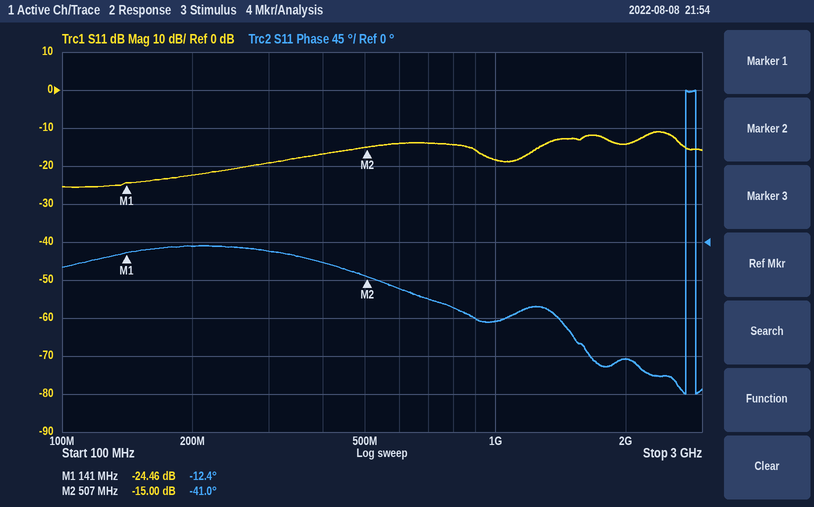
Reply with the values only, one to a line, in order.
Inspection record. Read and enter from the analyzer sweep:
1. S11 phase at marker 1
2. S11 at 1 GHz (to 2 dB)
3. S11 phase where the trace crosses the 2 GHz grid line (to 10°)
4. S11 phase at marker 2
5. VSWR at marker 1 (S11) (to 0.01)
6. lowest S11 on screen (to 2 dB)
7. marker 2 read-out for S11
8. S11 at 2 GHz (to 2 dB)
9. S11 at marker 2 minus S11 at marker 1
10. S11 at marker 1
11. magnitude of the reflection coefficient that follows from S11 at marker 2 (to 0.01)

-12.4°
-18 dB
-140°
-41.0°
1.13
-26 dB
-15.00 dB
-14 dB
9.46 dB
-24.46 dB
0.18
